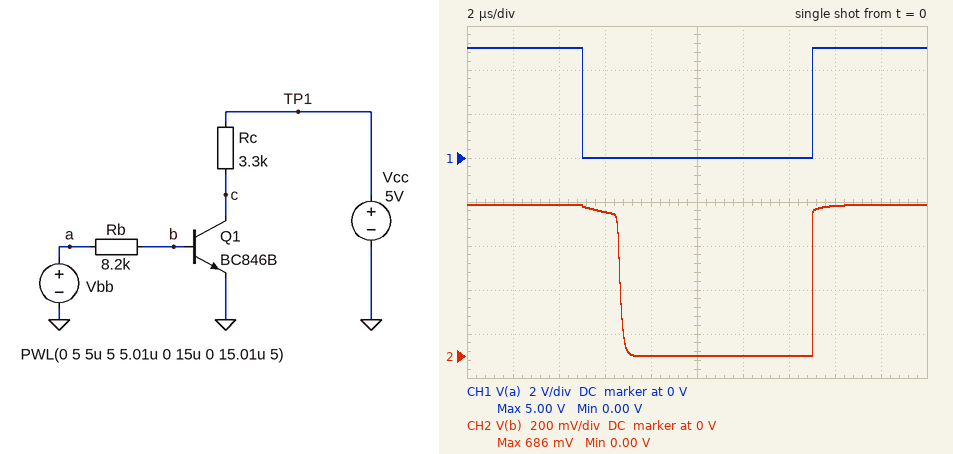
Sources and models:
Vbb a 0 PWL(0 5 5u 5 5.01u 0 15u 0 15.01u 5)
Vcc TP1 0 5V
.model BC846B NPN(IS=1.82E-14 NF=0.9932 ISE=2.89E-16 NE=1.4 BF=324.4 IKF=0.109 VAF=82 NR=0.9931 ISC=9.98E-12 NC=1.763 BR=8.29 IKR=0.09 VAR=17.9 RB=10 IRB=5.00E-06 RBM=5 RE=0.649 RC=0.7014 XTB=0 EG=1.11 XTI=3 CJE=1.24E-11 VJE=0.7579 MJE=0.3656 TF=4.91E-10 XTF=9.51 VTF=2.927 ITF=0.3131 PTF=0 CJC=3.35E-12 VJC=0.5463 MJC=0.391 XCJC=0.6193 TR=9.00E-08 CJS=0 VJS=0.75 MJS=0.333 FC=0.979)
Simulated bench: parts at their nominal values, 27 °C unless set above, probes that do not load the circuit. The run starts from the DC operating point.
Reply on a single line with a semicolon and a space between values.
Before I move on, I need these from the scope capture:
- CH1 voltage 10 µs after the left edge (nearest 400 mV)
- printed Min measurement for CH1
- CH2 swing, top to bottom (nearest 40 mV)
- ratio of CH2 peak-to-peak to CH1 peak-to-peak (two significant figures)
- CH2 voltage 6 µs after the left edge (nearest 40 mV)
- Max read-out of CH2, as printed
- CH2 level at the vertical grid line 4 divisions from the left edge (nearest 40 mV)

0 V; 0.00 V; 680 mV; 0.14; 640 mV; 686 mV; 0 V
